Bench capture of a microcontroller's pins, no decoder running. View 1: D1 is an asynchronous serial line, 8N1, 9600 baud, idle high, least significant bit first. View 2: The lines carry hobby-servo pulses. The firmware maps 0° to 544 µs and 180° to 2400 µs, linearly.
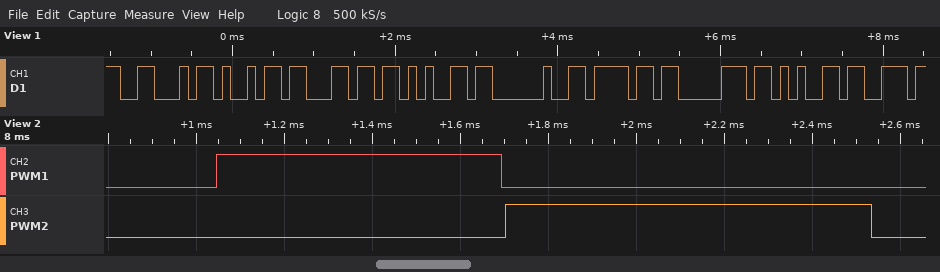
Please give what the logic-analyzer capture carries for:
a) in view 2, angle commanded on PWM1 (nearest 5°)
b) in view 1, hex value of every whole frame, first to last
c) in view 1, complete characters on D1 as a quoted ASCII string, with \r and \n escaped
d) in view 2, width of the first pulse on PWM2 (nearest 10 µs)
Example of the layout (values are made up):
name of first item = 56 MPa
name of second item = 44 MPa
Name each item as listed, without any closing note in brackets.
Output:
in view 2, angle commanded on PWM1 = 10°
in view 1, hex value of every whole frame, first to last = 46 69 6C 65 20 6F 70 65
in view 1, complete characters on D1 as a quoted ASCII string, with \r and \n escaped = "File ope"
in view 2, width of the first pulse on PWM2 = 830 µs
